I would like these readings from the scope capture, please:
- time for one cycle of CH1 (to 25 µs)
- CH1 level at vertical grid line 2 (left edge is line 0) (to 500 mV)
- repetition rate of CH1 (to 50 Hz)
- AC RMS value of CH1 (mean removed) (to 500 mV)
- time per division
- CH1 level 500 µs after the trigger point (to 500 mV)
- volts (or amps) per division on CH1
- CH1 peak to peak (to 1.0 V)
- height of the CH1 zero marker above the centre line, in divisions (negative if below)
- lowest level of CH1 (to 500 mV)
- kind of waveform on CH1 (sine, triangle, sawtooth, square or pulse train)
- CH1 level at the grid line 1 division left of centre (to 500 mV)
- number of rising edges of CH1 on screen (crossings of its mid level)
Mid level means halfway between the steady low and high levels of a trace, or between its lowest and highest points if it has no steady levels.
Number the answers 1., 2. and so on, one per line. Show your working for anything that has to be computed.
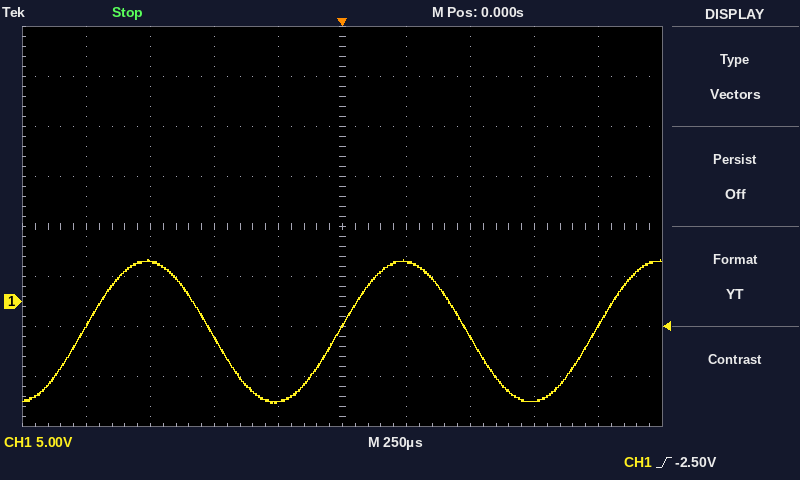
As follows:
1. 1.000 ms
2. 4.0 V
3. 1 / 1.000 ms ≈ 1.00 kHz
4. 14.0 V / (2√2) ≈ 5.0 V
5. 250 µs
6. -3.5 V
7. 5 V
8. 14.0 V
9. -1.5 div
10. -10.0 V
11. sine
12. -10.0 V
13. 3
